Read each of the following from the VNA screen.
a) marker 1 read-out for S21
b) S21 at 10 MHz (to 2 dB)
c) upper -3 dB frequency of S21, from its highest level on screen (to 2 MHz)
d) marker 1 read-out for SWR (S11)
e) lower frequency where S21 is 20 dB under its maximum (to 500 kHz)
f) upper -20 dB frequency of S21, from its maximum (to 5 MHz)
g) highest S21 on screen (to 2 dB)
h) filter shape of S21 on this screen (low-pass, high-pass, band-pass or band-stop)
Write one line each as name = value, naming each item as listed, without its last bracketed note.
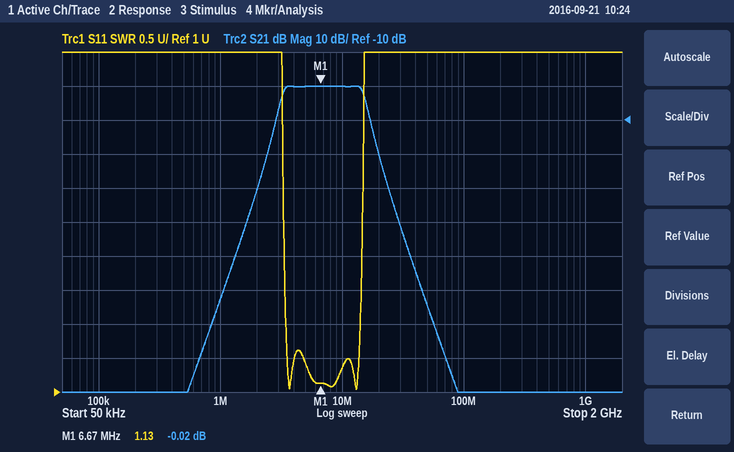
marker 1 read-out for S21 = -0.02 dB
S21 at 10 MHz = 0 dB
upper -3 dB frequency of S21, from its highest level on screen = 16 MHz
marker 1 read-out for SWR = 1.13
lower frequency where S21 is 20 dB under its maximum = 2.5 MHz
upper -20 dB frequency of S21, from its maximum = 20 MHz
highest S21 on screen = 0 dB
filter shape of S21 on this screen = band-pass
